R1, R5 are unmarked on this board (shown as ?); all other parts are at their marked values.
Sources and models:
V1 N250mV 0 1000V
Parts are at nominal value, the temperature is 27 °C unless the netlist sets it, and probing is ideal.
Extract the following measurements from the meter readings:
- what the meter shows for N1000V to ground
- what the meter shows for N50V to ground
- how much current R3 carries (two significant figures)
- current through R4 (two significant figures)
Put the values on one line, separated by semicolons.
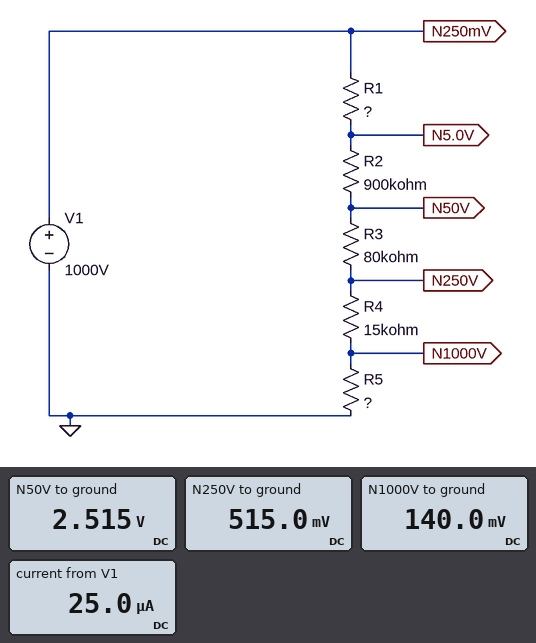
140.0 mV; 2.515 V; 25 µA; 25 µA
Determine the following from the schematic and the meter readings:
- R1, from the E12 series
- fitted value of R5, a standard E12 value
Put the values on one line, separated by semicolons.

39 MΩ; 5.6 kΩ
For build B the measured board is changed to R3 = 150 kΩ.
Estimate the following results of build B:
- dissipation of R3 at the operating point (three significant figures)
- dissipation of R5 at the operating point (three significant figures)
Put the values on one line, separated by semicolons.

93.4 µW; 3.49 µW
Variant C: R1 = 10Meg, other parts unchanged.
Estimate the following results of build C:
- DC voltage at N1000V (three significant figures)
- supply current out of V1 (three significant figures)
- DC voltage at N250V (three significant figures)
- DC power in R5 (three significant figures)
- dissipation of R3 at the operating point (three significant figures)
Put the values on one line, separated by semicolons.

509 mV; 90.9 µA; 1.87 V; 46.3 µW; 661 µW
